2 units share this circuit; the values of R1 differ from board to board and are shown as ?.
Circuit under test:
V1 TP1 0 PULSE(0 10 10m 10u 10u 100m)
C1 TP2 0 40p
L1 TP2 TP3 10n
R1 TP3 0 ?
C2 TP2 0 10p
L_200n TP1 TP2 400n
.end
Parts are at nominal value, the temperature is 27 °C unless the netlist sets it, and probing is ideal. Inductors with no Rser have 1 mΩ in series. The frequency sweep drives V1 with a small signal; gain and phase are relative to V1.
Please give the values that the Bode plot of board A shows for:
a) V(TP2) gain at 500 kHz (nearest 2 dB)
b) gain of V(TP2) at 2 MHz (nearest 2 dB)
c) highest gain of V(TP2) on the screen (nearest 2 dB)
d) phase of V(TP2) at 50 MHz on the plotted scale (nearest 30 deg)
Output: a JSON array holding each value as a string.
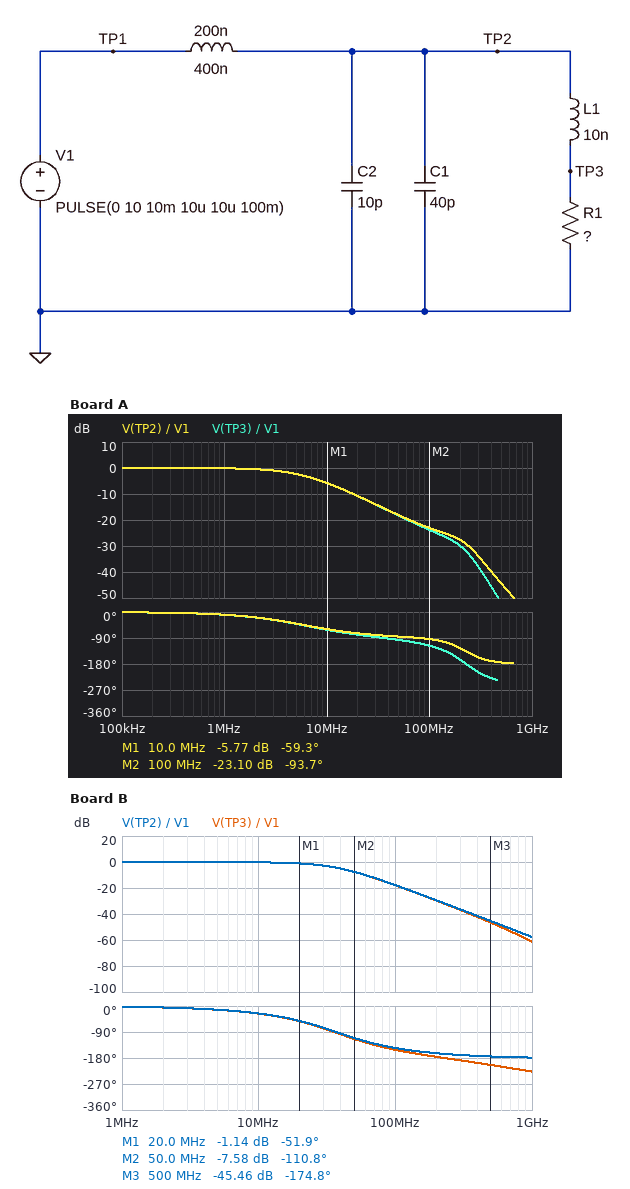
["0 dB", "0 dB", "0 dB", "-90 deg"]
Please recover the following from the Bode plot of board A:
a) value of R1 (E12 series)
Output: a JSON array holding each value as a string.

["15 Ω"]
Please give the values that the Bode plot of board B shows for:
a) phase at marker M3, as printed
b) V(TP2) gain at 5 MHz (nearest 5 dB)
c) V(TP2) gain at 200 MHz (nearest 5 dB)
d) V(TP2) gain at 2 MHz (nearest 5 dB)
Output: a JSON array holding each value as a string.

["-174.8 deg", "0 dB", "-30 dB", "0 dB"]
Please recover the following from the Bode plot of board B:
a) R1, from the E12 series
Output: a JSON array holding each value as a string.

["56 Ω"]
